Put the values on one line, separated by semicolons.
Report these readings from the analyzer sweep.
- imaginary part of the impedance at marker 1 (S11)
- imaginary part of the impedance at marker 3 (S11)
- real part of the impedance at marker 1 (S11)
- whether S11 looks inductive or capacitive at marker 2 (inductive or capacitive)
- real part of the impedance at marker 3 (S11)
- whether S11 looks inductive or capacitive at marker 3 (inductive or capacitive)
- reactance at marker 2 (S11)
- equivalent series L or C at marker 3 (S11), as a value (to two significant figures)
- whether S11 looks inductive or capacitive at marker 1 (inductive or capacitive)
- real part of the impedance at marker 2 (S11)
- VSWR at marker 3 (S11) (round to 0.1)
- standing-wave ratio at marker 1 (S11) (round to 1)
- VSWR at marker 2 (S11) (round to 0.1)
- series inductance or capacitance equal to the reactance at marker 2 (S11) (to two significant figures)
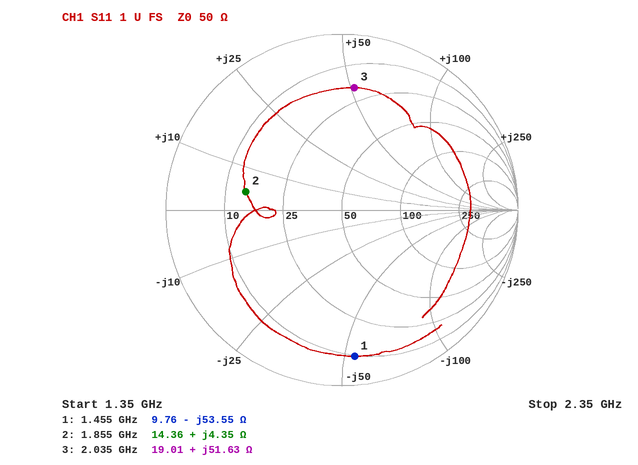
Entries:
-53.55 Ω; +51.63 Ω; 9.76 Ω; inductive; 19.01 Ω; inductive; +4.35 Ω; 4.0 nH; capacitive; 14.36 Ω; 5.6; 11; 3.5; 370 pH
